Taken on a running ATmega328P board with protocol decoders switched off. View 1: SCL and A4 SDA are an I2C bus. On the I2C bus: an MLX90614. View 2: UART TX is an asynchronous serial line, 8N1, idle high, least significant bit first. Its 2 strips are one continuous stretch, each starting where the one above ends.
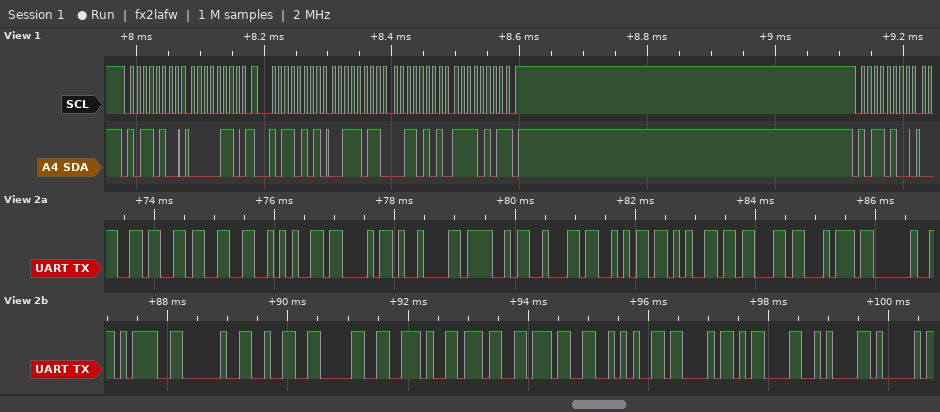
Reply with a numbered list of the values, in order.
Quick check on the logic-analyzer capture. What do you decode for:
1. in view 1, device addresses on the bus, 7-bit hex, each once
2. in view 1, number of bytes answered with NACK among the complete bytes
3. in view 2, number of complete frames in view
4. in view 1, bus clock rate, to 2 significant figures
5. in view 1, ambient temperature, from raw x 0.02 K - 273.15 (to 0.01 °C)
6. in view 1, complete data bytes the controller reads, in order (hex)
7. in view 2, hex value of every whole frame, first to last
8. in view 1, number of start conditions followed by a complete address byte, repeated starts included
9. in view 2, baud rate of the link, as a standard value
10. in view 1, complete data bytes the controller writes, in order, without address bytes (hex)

1. 0x5A
2. 1
3. 24
4. 100 kHz
5. -0.61 °C
6. 3B 35 F5
7. 36 33 2A 43 09 4F 62 6A 65 63 74 20 3D 20 32 30 2E 37 37 2A 43 0D 0A 41
8. 3
9. 9600 baud
10. 06
